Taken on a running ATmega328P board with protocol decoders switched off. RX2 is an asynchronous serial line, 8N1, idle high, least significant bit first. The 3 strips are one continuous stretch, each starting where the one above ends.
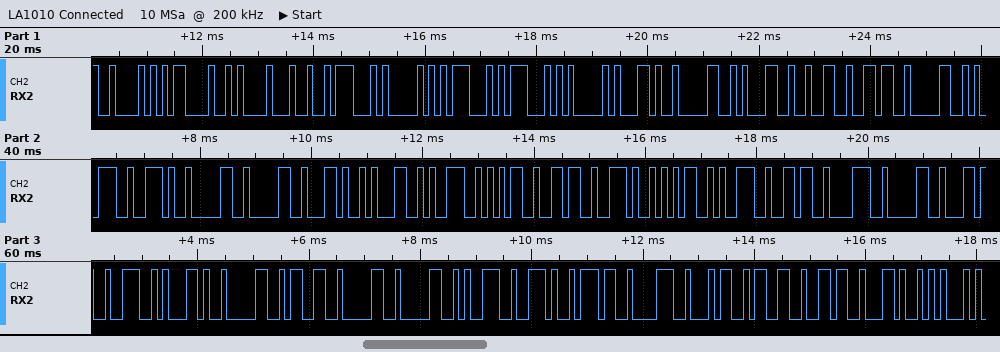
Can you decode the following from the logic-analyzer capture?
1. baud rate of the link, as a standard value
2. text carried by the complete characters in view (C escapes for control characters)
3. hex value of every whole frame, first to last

9600 baud
"B\r\n$GPGGA,012609.00,1956.59680,N,03009.78436,E"
42 0D 0A 24 47 50 47 47 41 2C 30 31 32 36 30 39 2E 30 30 2C 31 39 35 36 2E 35 39 36 38 30 2C 4E 2C 30 33 30 30 39 2E 37 38 34 33 36 2C 45
